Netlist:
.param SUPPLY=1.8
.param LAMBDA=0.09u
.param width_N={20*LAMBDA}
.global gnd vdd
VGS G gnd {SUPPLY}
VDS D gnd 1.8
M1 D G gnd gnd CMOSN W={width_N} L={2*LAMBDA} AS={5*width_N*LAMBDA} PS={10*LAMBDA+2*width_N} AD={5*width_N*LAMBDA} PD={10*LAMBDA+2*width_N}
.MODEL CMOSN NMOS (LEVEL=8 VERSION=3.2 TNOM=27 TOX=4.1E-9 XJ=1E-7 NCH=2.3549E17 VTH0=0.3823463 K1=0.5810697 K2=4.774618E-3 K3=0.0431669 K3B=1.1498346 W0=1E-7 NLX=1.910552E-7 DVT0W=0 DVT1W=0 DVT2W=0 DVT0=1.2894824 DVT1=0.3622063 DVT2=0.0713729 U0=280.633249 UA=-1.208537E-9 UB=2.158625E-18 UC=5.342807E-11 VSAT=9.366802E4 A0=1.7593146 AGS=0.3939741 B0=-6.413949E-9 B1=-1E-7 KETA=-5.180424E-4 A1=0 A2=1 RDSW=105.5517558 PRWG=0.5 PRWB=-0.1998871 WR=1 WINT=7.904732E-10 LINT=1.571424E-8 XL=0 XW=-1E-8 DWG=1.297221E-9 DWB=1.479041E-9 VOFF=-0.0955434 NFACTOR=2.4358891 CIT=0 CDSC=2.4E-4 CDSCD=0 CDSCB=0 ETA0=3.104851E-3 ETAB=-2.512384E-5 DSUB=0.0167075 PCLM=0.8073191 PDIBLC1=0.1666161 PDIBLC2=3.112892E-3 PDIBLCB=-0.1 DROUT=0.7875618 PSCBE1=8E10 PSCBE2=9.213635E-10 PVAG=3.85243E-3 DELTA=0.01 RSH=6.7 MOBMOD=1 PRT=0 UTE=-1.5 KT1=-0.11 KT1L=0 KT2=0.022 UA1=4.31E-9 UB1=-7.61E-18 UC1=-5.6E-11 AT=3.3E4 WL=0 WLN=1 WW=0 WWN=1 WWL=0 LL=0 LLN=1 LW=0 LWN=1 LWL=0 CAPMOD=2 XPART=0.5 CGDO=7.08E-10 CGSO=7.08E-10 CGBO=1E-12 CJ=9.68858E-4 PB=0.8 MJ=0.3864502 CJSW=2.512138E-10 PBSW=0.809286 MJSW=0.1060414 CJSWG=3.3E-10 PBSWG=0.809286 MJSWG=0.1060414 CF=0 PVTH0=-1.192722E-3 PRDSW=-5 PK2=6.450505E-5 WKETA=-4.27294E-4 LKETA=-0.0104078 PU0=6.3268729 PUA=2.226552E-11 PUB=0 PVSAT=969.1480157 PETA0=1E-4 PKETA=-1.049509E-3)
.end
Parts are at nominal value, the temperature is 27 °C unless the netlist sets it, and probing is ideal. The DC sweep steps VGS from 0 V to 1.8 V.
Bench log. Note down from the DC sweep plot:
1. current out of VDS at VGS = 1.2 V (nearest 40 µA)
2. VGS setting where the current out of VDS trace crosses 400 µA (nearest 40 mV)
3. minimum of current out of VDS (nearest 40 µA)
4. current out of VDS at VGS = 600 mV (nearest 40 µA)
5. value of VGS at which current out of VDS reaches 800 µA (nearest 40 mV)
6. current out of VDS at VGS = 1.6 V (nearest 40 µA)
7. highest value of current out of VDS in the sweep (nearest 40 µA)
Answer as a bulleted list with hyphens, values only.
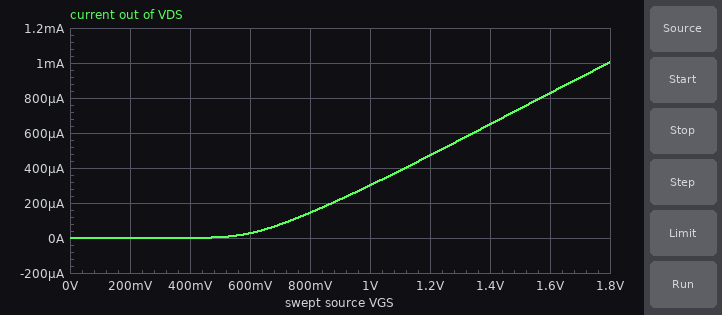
- 480 µA
- 1.12 V
- 0 A
- 40 µA
- 1.56 V
- 840 µA
- 1.00 mA
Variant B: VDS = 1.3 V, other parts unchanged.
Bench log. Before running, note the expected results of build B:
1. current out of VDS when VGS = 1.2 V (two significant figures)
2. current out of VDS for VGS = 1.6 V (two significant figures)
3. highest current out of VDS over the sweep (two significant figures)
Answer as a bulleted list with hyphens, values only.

- 450 µA
- 800 µA
- 980 µA
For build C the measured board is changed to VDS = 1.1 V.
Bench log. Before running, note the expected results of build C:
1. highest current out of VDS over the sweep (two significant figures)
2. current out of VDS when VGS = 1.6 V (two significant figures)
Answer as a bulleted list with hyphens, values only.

- 960 µA
- 790 µA
